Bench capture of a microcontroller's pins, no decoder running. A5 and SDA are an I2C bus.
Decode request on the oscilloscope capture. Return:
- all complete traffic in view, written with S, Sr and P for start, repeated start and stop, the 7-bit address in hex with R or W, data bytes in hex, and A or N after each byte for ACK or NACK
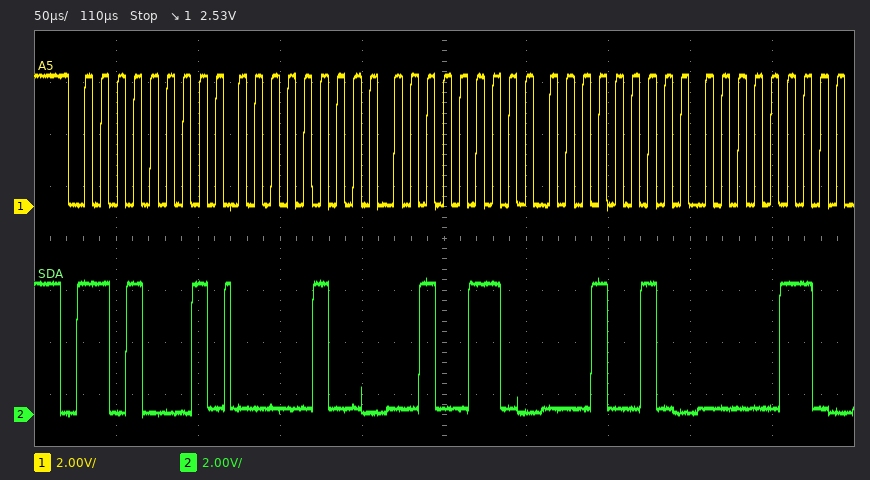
S 68R A 04 A 26 A 12 A 06 A
